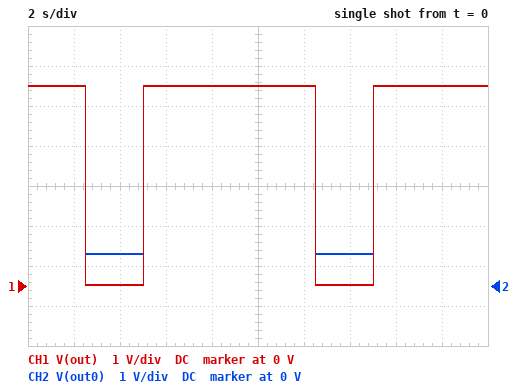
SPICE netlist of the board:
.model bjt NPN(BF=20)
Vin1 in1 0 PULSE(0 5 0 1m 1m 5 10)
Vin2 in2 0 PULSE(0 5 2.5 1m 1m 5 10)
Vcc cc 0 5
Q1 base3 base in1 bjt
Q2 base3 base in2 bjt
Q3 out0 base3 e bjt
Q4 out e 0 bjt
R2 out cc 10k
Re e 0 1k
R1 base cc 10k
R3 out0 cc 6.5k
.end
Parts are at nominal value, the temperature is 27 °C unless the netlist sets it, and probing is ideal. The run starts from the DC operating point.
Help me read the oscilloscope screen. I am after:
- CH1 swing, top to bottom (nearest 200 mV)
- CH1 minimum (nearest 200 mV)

5.0 V
0 V
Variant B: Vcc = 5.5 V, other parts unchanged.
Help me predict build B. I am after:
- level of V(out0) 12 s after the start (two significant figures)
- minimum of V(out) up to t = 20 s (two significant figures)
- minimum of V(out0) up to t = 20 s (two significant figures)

5.5 V
29 mV
820 mV
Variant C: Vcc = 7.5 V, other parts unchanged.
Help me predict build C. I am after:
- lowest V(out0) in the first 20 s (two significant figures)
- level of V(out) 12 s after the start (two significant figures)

830 mV
7.5 V
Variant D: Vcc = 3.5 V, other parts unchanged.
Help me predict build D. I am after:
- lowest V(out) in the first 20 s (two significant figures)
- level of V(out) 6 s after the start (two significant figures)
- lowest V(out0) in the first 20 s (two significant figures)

3.1 V
3.5 V
720 mV
